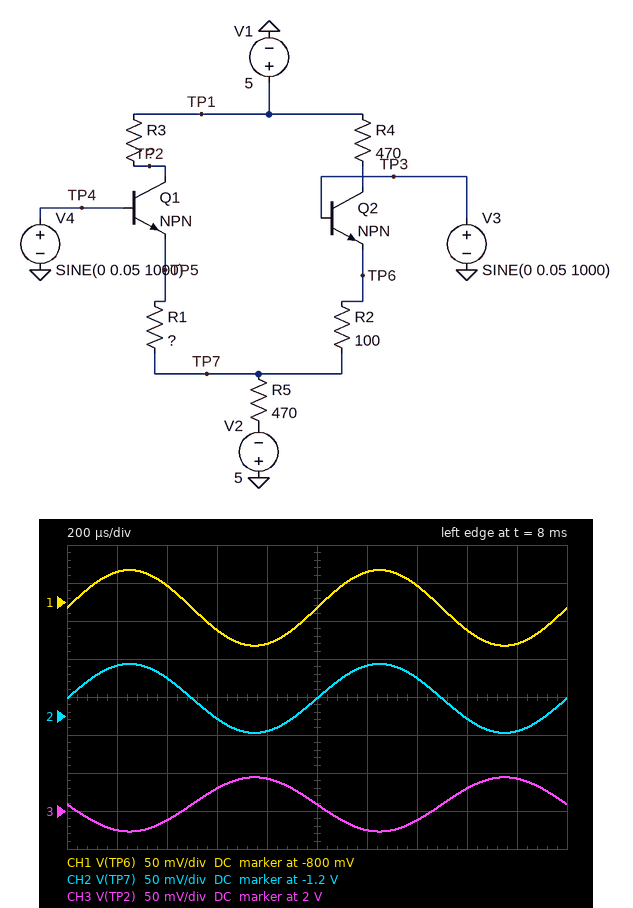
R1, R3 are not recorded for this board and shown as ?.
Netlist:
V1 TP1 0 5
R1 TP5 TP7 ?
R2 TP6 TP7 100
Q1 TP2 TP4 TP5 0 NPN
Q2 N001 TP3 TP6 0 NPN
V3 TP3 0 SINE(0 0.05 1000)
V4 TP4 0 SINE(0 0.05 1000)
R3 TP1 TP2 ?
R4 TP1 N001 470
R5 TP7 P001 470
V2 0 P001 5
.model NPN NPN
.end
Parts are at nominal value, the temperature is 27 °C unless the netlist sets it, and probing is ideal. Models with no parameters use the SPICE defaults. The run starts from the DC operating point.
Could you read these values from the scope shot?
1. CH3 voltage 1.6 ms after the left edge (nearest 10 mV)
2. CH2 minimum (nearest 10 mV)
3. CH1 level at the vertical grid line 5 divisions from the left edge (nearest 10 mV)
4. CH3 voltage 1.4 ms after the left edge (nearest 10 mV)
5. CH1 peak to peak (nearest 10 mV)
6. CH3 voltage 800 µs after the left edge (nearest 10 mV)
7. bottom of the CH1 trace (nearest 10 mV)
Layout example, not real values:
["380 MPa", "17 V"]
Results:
["2.03 V", "-1.22 V", "-810 mV", "1.99 V", "100 mV", "2.04 V", "-860 mV"]
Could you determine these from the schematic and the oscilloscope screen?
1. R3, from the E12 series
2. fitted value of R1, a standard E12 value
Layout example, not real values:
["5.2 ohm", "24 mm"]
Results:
["680 Ω", "82 Ω"]
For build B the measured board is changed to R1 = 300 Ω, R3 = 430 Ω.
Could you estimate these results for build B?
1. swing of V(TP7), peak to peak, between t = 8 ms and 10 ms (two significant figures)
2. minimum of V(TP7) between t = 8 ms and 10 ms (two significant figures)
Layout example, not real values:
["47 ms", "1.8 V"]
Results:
["86 mV", "-1.4 V"]
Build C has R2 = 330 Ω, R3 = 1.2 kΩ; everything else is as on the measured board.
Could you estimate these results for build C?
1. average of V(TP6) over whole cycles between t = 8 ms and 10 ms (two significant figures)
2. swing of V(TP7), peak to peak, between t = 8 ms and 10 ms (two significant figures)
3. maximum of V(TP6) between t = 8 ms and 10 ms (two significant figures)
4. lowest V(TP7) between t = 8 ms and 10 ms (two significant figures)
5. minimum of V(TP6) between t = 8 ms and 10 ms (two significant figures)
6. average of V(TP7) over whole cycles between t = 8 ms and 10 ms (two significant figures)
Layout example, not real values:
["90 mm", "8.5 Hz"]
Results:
["-790 mV", "87 mV", "-740 mV", "-1.4 V", "-840 mV", "-1.3 V"]
